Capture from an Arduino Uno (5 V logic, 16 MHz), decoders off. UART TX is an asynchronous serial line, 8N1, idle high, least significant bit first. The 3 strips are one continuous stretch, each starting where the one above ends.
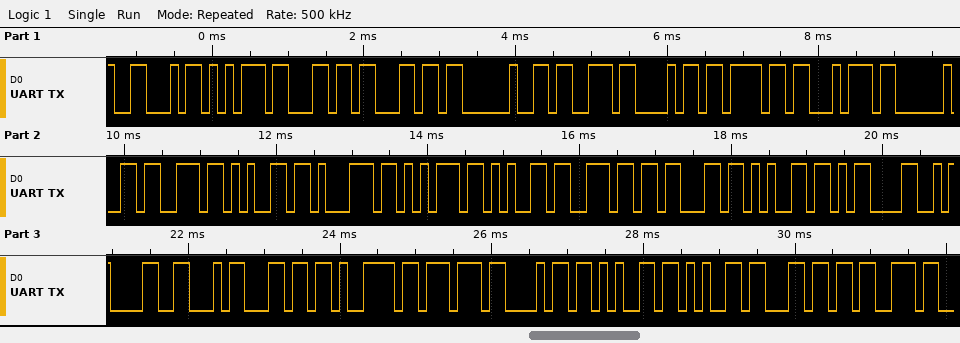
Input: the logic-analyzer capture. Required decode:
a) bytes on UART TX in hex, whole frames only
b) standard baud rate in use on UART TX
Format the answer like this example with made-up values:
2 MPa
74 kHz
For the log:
0x46 0x75 0x6C 0x6C 0x20 0x73 0x68 0x6F 0x74 0x20 0x73 0x65 0x71 0x75 0x65 0x6E 0x63 0x65 0x0D 0x0A 0x46 0x6C 0x79 0x77 0x68 0x65 0x65 0x6C 0x73
9600 baud
